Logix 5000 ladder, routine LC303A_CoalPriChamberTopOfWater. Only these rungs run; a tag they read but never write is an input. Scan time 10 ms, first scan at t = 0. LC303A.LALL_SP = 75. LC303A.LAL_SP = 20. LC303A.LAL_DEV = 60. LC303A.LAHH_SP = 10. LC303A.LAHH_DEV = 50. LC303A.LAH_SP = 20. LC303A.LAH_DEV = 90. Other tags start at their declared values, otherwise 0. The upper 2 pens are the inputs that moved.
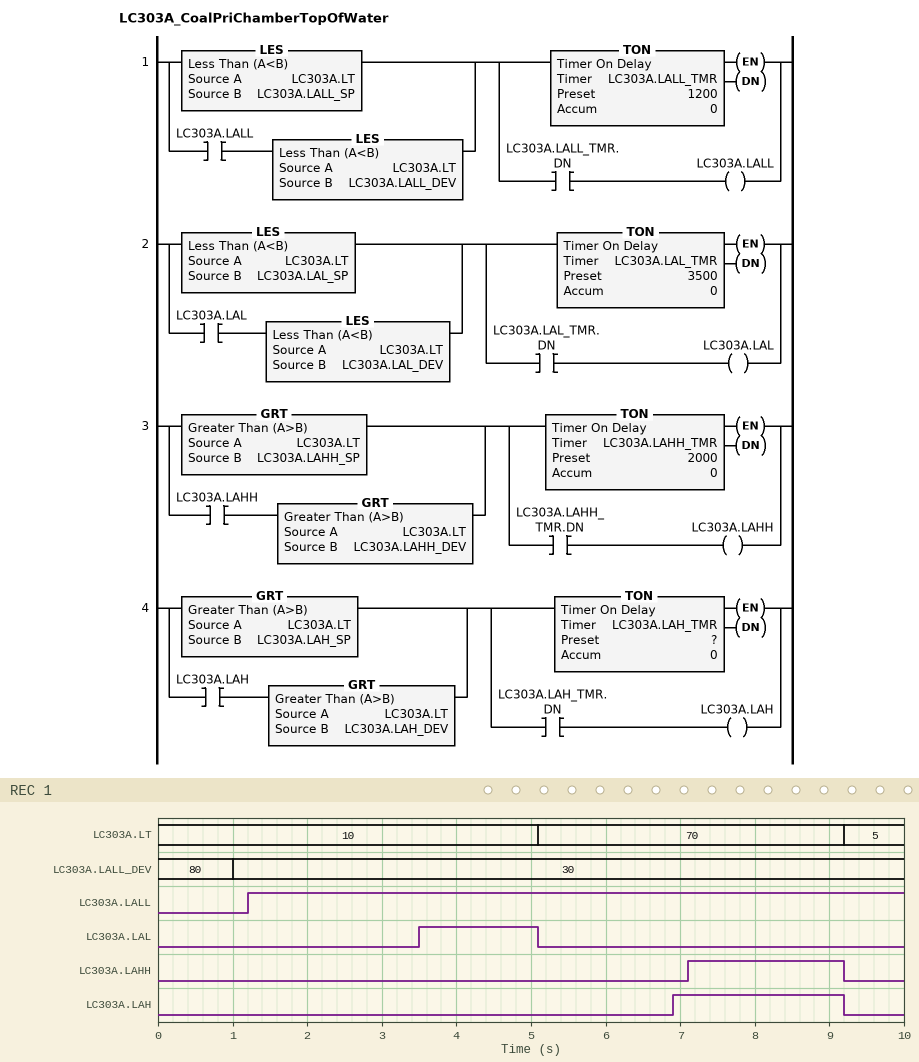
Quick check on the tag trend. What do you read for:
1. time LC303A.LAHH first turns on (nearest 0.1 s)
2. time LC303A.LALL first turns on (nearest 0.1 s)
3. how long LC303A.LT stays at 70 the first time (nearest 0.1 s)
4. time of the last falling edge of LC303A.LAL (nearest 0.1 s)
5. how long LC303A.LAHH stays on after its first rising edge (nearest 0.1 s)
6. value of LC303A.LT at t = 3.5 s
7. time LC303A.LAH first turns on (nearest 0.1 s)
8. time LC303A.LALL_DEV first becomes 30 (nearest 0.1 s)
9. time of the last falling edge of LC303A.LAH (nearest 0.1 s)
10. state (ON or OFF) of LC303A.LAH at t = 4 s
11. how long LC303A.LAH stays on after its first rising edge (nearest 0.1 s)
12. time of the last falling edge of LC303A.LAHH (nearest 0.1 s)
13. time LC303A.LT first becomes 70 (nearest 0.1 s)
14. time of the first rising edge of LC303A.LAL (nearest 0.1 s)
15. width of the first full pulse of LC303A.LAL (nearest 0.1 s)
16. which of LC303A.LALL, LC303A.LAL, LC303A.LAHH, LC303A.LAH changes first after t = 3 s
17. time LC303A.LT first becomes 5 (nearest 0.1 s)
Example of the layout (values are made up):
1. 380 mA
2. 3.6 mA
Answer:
1. 7.1 s
2. 1.2 s
3. 4.1 s
4. 5.1 s
5. 2.1 s
6. 10
7. 6.9 s
8. 1.0 s
9. 9.2 s
10. OFF
11. 2.3 s
12. 9.2 s
13. 5.1 s
14. 3.5 s
15. 1.6 s
16. LC303A.LAL
17. 9.2 s
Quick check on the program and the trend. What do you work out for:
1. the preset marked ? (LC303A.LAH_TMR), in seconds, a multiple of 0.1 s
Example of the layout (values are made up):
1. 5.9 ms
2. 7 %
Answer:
1. 1.8 s
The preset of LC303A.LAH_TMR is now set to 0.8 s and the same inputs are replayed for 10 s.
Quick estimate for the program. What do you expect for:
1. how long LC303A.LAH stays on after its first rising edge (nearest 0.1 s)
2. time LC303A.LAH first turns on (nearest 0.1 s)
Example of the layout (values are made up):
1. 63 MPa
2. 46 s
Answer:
1. 3.3 s
2. 5.9 s
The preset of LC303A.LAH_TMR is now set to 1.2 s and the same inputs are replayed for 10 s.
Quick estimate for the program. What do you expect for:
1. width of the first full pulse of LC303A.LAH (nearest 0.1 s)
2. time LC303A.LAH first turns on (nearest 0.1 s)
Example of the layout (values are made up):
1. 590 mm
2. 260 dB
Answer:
1. 2.9 s
2. 6.3 s
